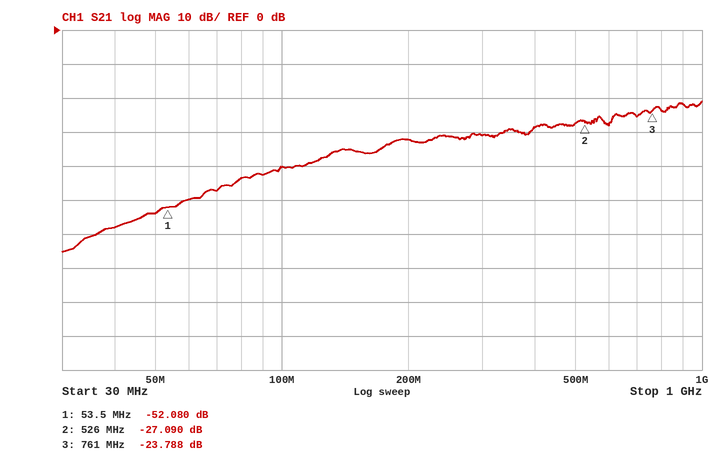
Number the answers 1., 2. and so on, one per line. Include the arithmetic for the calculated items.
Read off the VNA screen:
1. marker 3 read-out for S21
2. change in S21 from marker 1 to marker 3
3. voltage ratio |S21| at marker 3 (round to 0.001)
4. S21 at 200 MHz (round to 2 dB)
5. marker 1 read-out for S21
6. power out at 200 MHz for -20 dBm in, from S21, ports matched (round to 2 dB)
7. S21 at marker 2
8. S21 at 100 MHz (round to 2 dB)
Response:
1. -23.788 dB
2. -23.788 − (-52.08) = 28.292 dB
3. 10^(-23.788/20) ≈ 0.065
4. -32 dB
5. -52.080 dB
6. -20 dBm + (-32 dB) = -52 dBm
7. -27.090 dB
8. -40 dB
